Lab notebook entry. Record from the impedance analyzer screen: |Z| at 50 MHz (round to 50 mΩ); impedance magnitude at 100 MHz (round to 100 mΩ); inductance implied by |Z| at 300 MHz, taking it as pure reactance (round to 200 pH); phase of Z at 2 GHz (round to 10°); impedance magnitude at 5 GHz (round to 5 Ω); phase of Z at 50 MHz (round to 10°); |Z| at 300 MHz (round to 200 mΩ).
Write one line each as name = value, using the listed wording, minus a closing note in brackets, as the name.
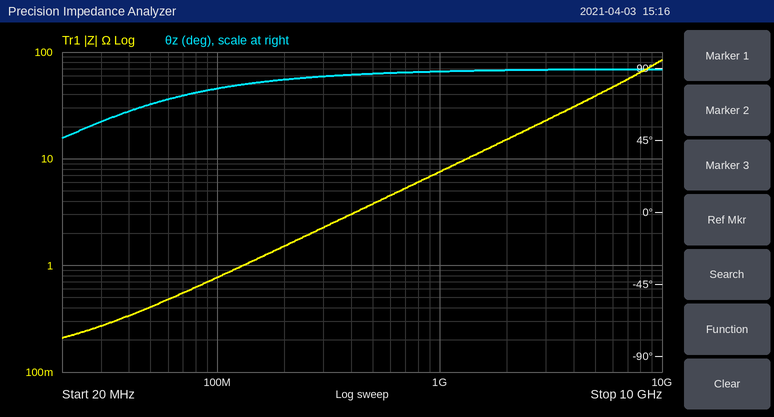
|Z| at 50 MHz = 400 mΩ
impedance magnitude at 100 MHz = 800 mΩ
inductance implied by |Z| at 300 MHz, taking it as pure reactance = 1.2 nH
phase of Z at 2 GHz = 90°
impedance magnitude at 5 GHz = 40 Ω
phase of Z at 50 MHz = 70°
|Z| at 300 MHz = 2.2 Ω
